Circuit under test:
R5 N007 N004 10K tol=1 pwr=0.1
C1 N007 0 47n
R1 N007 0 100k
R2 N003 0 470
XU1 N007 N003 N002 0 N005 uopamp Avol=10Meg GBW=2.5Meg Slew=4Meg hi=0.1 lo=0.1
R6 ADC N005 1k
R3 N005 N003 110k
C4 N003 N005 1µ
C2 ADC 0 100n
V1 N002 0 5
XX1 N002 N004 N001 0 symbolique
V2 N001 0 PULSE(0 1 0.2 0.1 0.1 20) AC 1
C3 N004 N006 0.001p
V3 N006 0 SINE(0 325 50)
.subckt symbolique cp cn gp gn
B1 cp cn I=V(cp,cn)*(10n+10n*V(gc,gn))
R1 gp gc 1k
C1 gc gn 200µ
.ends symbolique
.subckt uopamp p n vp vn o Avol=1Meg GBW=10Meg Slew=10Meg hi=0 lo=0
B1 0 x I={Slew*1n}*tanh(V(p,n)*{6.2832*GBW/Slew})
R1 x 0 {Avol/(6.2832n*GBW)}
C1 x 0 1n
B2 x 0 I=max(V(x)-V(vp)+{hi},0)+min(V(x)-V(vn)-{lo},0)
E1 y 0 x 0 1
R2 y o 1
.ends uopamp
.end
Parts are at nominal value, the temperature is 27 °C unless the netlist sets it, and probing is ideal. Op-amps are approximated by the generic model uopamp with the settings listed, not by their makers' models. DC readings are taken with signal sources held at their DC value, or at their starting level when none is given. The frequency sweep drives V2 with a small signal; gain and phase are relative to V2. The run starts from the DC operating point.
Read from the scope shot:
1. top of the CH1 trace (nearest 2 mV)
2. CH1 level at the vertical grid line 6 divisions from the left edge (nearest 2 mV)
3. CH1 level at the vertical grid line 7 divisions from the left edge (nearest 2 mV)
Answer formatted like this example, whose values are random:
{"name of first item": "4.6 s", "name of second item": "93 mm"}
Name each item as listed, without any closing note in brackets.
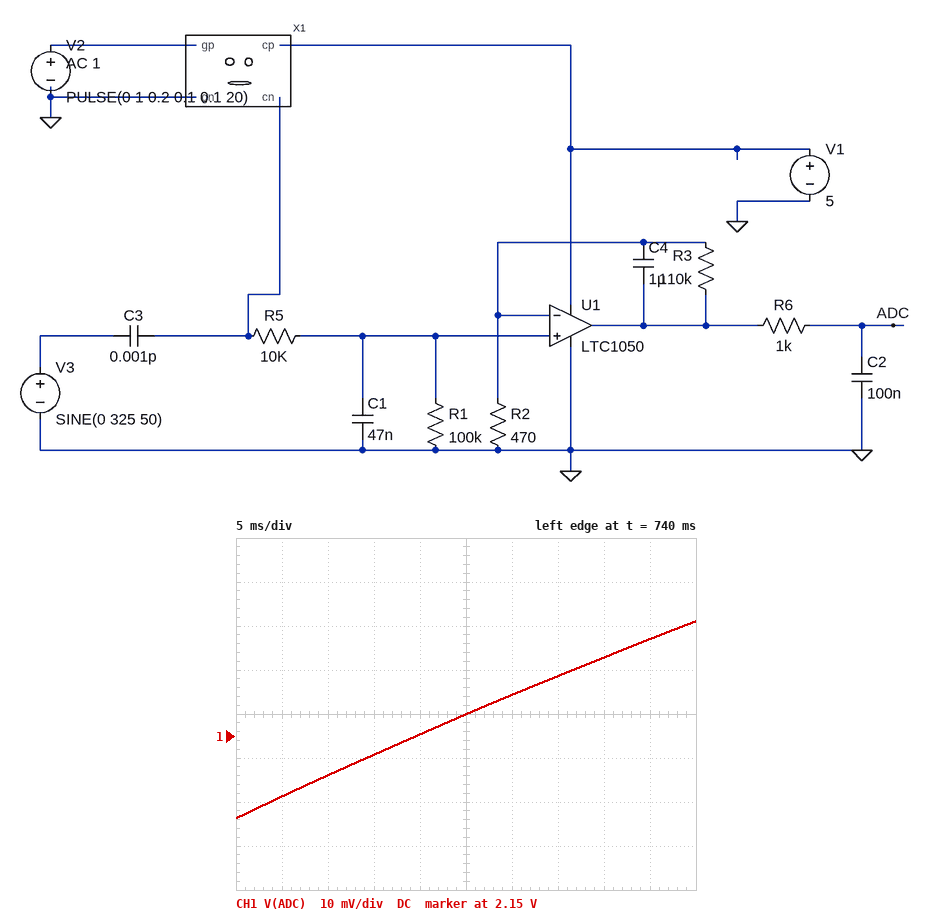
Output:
{"top of the CH1 trace": "2.176 V", "CH1 level at the vertical grid line 6 divisions from the left edge": "2.160 V", "CH1 level at the vertical grid line 7 divisions from the left edge": "2.164 V"}
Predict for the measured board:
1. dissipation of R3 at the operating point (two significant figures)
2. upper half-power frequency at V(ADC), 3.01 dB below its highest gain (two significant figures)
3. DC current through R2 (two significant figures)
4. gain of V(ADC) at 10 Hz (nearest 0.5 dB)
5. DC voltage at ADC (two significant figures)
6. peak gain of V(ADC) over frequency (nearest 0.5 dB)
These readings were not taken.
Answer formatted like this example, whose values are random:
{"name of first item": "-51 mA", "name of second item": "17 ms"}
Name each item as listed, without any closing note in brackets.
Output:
{"dissipation of R3 at the operating point": "12 µW", "upper half-power frequency at V(ADC), 3.01 dB below its highest gain": "650 mHz", "DC current through R2": "11 µA", "gain of V(ADC) at 10 Hz": "-38.0 dB", "DC voltage at ADC": "1.2 V", "peak gain of V(ADC) over frequency": "1.5 dB"}
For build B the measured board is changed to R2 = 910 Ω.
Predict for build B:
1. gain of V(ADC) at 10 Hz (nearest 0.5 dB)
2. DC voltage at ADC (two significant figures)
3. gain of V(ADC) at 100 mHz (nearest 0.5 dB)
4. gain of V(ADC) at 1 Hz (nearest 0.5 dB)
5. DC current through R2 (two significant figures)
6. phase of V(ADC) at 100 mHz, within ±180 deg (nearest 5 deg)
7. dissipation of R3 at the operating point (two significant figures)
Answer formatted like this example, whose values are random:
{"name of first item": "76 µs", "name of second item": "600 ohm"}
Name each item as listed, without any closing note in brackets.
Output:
{"gain of V(ADC) at 10 Hz": "-43.5 dB", "DC voltage at ADC": "610 mV", "gain of V(ADC) at 100 mHz": "-4.5 dB", "gain of V(ADC) at 1 Hz": "-10.0 dB", "DC current through R2": "5.5 µA", "phase of V(ADC) at 100 mHz, within ±180 deg": "-10 deg", "dissipation of R3 at the operating point": "3.3 µW"}
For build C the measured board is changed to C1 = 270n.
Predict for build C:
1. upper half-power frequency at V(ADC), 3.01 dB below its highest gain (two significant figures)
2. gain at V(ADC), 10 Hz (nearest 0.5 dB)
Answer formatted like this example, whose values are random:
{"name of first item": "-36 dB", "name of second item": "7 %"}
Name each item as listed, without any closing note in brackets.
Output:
{"upper half-power frequency at V(ADC), 3.01 dB below its highest gain": "640 mHz", "gain at V(ADC), 10 Hz": "-43.5 dB"}
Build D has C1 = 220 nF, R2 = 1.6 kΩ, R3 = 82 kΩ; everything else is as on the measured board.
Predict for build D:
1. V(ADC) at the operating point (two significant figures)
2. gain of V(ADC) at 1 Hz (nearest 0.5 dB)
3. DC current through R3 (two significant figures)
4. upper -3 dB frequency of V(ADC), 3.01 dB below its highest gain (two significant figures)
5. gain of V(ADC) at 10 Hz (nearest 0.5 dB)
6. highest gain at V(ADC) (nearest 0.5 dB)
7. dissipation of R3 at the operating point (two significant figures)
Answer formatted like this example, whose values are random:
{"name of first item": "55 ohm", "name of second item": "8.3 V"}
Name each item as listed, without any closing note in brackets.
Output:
{"V(ADC) at the operating point": "260 mV", "gain of V(ADC) at 1 Hz": "-17.0 dB", "DC current through R3": "3.1 µA", "upper -3 dB frequency of V(ADC), 3.01 dB below its highest gain": "690 mHz", "gain of V(ADC) at 10 Hz": "-52.5 dB", "highest gain at V(ADC)": "-11.5 dB", "dissipation of R3 at the operating point": "800 nW"}
